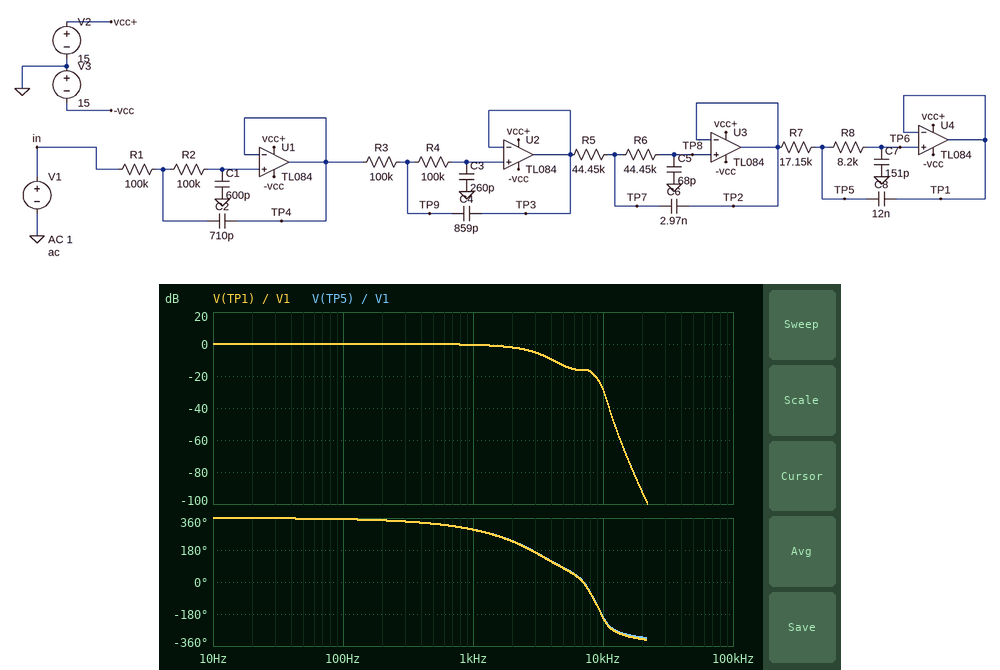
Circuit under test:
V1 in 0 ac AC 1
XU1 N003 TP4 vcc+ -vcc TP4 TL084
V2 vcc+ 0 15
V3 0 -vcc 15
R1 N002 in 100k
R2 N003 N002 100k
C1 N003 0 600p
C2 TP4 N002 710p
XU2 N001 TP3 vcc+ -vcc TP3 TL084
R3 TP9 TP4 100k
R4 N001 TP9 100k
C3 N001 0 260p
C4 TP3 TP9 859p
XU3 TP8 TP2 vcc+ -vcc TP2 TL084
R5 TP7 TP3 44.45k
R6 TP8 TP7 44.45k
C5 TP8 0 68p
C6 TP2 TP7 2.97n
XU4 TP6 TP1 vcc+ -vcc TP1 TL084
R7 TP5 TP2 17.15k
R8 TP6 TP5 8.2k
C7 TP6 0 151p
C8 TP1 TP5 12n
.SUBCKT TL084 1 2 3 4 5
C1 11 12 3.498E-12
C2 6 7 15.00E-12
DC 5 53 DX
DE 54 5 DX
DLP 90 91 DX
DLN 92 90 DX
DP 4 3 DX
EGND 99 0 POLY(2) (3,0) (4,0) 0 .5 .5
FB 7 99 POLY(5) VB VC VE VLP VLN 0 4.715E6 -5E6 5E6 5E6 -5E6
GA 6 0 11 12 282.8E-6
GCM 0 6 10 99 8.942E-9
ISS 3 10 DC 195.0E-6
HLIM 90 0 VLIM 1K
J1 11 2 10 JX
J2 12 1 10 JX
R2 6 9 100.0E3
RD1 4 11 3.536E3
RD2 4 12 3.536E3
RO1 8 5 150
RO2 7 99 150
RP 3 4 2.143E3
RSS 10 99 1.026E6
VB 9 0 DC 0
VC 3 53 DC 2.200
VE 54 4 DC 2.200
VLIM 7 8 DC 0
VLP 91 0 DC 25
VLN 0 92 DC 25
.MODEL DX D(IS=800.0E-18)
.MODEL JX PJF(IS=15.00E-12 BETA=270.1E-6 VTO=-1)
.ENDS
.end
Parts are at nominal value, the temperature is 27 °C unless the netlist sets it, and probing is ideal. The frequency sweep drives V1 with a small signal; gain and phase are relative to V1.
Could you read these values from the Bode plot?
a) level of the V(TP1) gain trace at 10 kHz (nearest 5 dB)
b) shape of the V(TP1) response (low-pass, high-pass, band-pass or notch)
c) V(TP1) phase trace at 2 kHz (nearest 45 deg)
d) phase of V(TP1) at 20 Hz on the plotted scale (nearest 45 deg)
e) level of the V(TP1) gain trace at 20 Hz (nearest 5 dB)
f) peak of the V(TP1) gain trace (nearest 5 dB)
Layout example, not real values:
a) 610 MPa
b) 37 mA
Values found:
a) -30 dB
b) low-pass
c) 225 deg
d) 360 deg
e) 0 dB
f) 0 dB
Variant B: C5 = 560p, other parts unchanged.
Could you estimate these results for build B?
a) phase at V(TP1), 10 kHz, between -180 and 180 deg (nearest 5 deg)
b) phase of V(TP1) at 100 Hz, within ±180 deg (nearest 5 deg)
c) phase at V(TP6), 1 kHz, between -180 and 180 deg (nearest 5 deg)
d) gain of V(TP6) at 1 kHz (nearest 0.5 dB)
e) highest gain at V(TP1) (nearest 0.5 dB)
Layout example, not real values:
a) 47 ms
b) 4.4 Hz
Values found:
a) 140 deg
b) -10 deg
c) -85 deg
d) 0 dB
e) 0 dB
